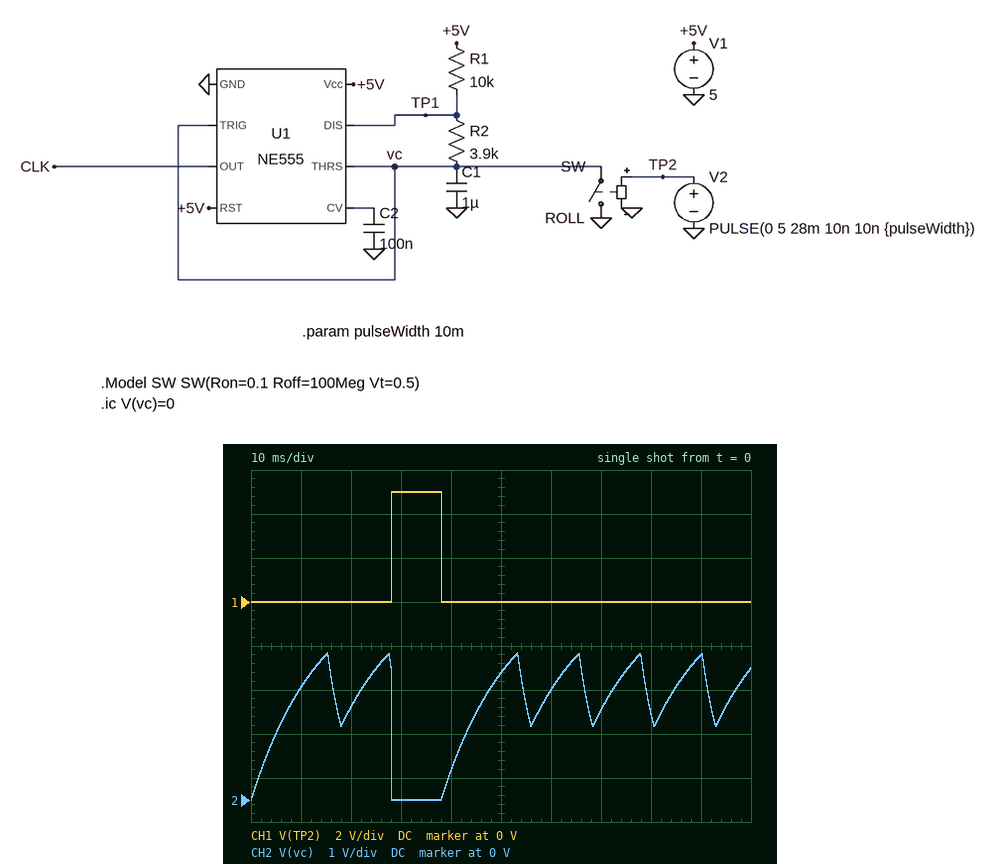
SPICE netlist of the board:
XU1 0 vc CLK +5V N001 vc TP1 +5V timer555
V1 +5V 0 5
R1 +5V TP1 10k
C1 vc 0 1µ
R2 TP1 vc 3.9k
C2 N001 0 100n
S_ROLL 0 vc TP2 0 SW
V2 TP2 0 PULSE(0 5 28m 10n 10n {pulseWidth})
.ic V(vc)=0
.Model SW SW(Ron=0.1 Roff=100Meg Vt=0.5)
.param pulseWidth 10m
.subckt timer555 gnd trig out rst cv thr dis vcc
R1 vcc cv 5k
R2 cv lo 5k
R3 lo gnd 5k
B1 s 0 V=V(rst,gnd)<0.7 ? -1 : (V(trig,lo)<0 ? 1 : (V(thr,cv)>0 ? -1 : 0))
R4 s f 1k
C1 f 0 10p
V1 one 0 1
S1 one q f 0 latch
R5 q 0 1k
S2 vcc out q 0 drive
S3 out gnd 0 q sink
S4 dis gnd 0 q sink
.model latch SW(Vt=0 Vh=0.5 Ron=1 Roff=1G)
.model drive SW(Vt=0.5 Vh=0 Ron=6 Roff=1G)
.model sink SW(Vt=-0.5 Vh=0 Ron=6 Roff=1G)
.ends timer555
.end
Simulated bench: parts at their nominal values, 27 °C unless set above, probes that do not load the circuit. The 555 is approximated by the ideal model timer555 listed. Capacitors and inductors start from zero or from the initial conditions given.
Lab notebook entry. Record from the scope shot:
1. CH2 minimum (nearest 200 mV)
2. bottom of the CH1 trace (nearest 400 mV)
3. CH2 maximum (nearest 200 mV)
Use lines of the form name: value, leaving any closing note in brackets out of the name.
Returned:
CH2 minimum: 0 V
bottom of the CH1 trace: 0 V
CH2 maximum: 3.4 V
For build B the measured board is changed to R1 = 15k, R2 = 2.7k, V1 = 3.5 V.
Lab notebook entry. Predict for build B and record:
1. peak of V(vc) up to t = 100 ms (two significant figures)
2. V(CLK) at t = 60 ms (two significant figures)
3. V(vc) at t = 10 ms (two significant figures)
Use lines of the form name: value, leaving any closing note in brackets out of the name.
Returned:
peak of V(vc) up to t = 100 ms: 2.3 V
V(CLK) at t = 60 ms: 3.5 V
V(vc) at t = 10 ms: 1.5 V
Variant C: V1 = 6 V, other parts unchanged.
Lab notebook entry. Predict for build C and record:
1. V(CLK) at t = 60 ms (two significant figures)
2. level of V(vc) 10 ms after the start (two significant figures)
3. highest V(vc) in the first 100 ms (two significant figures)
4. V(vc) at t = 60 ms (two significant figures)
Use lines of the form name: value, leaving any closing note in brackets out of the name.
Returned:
V(CLK) at t = 60 ms: 6.0 V
level of V(vc) 10 ms after the start: 3.1 V
highest V(vc) in the first 100 ms: 4.0 V
V(vc) at t = 60 ms: 3.0 V
